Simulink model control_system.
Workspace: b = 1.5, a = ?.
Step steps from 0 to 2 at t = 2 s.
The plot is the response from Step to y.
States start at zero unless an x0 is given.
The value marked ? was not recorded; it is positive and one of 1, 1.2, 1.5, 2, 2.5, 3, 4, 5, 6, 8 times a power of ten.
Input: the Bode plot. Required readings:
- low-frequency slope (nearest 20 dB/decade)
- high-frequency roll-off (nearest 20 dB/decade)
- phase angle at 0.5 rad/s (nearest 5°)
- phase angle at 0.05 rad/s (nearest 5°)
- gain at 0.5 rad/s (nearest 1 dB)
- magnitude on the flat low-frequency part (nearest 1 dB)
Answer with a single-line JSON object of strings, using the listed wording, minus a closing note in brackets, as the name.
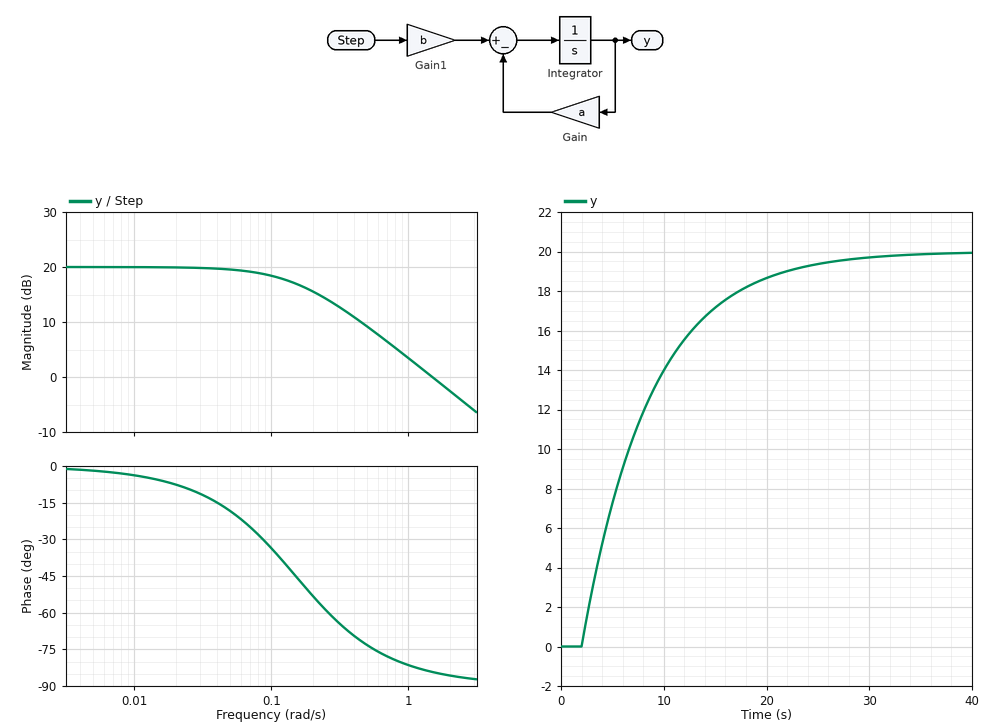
{"low-frequency slope": "0 dB/decade", "high-frequency roll-off": "-20 dB/decade", "phase angle at 0.5 rad/s": "-75°", "phase angle at 0.05 rad/s": "-20°", "gain at 0.5 rad/s": "9 dB", "magnitude on the flat low-frequency part": "20 dB"}
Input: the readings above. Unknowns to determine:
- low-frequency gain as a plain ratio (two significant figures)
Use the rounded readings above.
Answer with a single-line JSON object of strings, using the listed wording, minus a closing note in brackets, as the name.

{"low-frequency gain as a plain ratio": "10"}
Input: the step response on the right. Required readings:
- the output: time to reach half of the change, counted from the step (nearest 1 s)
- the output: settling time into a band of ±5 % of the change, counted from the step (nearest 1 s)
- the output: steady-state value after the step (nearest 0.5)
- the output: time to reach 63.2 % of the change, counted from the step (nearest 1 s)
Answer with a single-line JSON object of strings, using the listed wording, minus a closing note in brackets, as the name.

{"the output: time to reach half of the change, counted from the step": "5 s", "the output: settling time into a band of ±5 % of the change, counted from the step": "20 s", "the output: steady-state value after the step": "20.0", "the output: time to reach 63.2 % of the change, counted from the step": "7 s"}
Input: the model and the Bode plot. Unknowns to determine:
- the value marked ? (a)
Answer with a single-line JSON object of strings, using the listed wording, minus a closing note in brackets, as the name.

{"the value marked ?": "0.15"}
